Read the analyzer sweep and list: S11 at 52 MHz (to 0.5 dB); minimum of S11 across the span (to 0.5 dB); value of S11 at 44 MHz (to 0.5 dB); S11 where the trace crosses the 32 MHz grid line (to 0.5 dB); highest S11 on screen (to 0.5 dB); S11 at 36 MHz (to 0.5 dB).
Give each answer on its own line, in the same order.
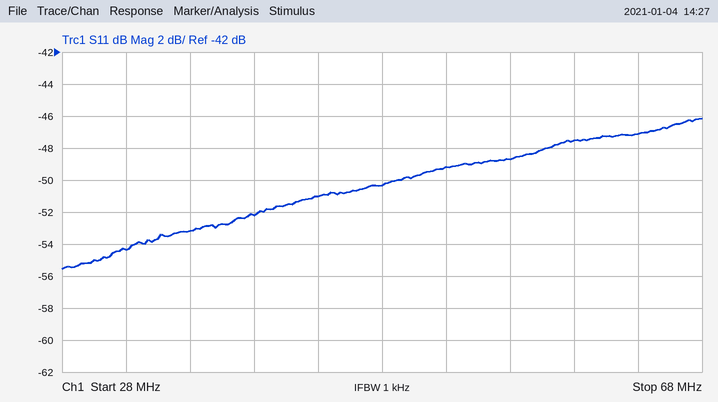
-49.0 dB
-55.5 dB
-51.0 dB
-54.5 dB
-46.0 dB
-53.0 dB
